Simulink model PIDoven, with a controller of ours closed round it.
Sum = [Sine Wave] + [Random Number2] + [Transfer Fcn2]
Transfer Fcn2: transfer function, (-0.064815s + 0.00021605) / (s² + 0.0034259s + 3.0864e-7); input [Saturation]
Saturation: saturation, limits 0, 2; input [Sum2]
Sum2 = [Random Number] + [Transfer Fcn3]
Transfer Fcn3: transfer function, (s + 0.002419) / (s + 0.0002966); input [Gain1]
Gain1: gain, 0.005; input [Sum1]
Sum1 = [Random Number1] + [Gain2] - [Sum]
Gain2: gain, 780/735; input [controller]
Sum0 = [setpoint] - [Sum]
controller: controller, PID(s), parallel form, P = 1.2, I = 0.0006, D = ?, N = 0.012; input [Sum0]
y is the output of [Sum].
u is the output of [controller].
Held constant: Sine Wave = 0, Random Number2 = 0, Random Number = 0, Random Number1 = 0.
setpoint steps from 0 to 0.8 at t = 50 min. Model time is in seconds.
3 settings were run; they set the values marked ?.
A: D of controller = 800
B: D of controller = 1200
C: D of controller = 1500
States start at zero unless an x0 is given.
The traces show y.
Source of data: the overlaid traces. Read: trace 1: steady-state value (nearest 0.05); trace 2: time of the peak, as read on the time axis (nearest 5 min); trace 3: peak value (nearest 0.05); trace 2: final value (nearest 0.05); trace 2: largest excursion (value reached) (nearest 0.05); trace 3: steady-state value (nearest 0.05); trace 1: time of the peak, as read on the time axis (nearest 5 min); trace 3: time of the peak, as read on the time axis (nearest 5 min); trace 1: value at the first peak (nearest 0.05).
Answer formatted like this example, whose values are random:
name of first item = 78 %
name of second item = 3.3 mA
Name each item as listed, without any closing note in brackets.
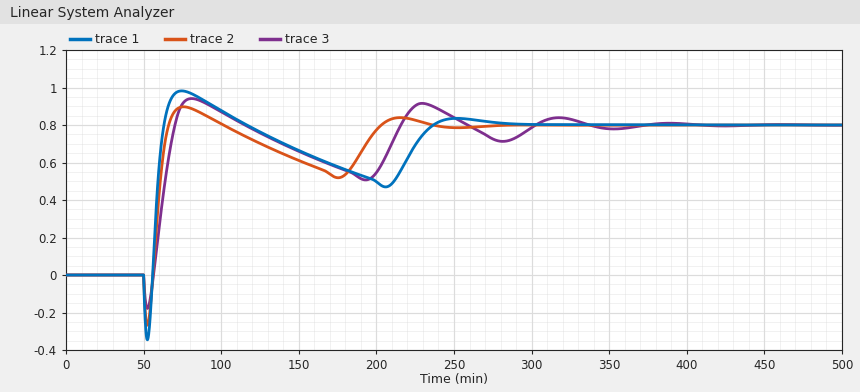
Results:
trace 1: steady-state value = 0.80
trace 2: time of the peak, as read on the time axis = 75 min
trace 3: peak value = 0.95
trace 2: final value = 0.80
trace 2: largest excursion (value reached) = 0.90
trace 3: steady-state value = 0.80
trace 1: time of the peak, as read on the time axis = 75 min
trace 3: time of the peak, as read on the time axis = 80 min
trace 1: value at the first peak = 1.00
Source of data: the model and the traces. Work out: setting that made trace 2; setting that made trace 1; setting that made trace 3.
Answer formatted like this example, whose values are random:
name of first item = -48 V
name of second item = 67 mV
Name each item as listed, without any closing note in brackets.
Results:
setting that made trace 2 = B
setting that made trace 1 = C
setting that made trace 3 = A
